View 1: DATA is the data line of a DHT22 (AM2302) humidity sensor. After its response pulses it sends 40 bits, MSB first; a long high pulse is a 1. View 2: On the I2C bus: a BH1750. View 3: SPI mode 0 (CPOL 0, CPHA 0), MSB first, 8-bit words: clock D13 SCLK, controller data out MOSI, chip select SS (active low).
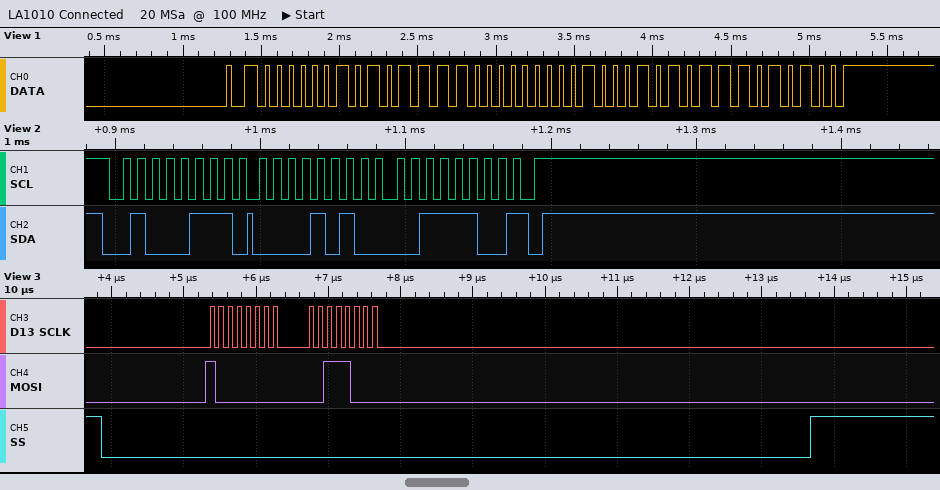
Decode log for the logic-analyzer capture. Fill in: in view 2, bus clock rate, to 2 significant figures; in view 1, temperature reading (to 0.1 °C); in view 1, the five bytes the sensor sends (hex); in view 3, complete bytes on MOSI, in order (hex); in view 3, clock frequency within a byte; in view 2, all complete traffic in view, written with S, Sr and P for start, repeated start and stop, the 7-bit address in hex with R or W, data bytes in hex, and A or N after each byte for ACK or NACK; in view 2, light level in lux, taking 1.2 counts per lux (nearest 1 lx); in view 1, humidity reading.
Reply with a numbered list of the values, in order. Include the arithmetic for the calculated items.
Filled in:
1. 100 kHz
2. 27.7 °C
3. 02 BC 01 15 D4
4. 0x80 0x38
5. 8 MHz
6. S 23R A 0A A 3C N P
7. 2620 / 1.2 = 2183 lx
8. 70.0 %
